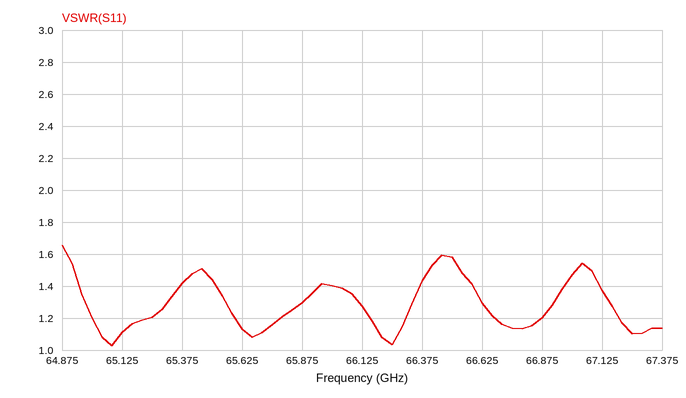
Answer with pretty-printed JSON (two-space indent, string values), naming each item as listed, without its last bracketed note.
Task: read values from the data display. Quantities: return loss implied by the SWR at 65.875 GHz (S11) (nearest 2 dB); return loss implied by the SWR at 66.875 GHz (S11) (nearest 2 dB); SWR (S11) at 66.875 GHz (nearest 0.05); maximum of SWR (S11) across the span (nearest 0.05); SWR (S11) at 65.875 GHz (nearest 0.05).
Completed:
{
  "return loss implied by the SWR at 65.875 GHz (S11)": "18 dB",
  "return loss implied by the SWR at 66.875 GHz (S11)": "20 dB",
  "SWR (S11) at 66.875 GHz": "1.20",
  "maximum of SWR (S11) across the span": "1.65",
  "SWR (S11) at 65.875 GHz": "1.30"
}
